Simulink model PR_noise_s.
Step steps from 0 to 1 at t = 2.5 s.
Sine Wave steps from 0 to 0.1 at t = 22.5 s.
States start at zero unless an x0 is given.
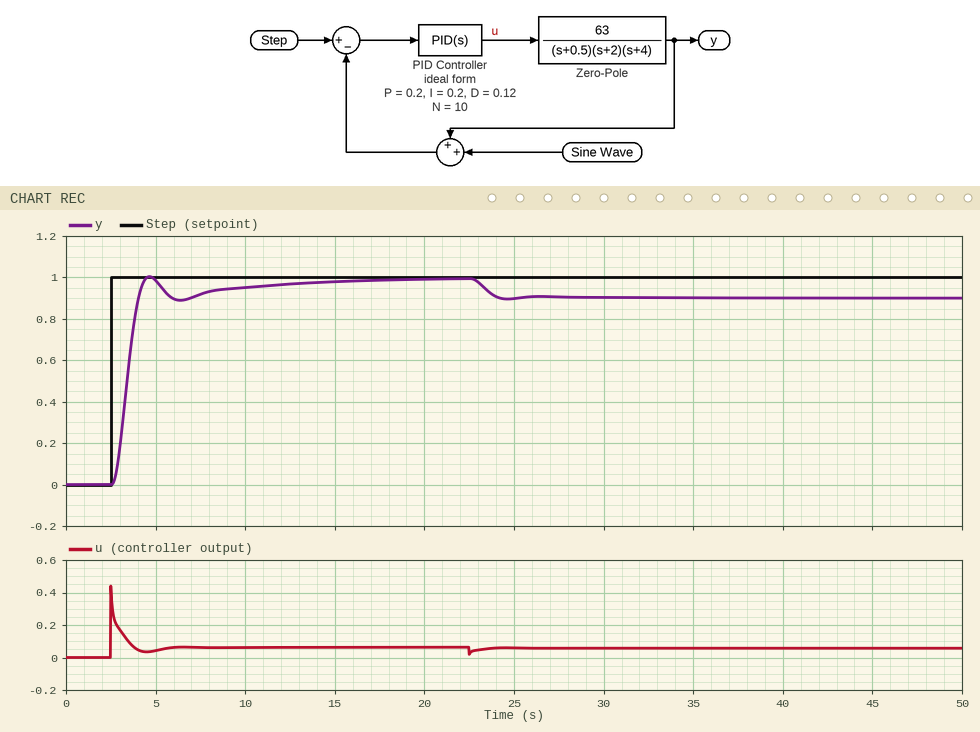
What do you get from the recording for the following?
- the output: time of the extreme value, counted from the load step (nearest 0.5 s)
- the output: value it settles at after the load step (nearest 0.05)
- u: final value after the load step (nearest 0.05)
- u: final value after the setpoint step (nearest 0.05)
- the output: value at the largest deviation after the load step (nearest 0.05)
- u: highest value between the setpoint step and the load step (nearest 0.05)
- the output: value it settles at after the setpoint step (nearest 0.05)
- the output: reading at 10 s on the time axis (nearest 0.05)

2.0 s
0.90
0.05
0.05
0.90
0.45
1.00
0.95
